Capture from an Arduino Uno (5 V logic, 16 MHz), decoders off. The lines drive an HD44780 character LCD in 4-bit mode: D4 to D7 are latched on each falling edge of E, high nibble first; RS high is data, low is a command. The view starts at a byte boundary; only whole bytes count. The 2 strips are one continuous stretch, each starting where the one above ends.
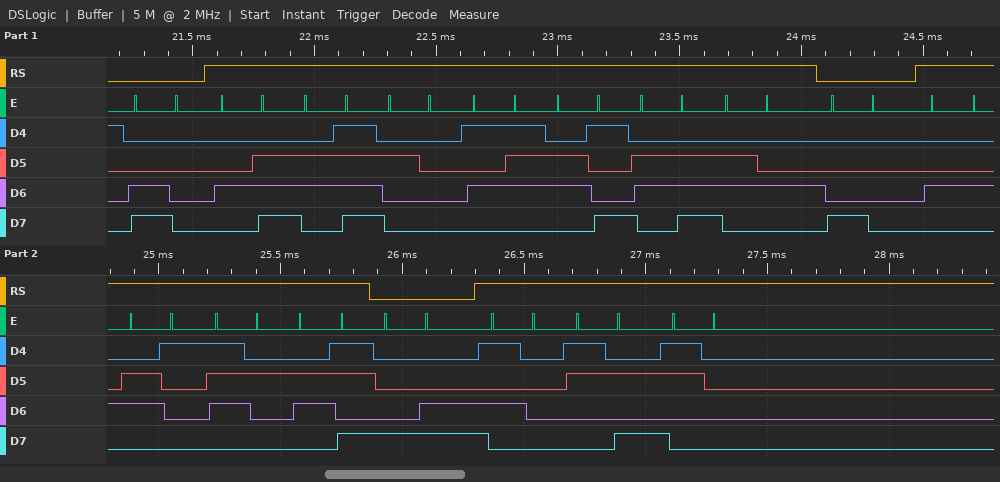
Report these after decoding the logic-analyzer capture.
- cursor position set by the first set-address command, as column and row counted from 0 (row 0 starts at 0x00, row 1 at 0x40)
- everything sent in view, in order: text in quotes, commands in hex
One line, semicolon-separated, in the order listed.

column 0, row 1; 0xC0 "No Wind" 0x80 "Dark" 0x8C "P:0"
